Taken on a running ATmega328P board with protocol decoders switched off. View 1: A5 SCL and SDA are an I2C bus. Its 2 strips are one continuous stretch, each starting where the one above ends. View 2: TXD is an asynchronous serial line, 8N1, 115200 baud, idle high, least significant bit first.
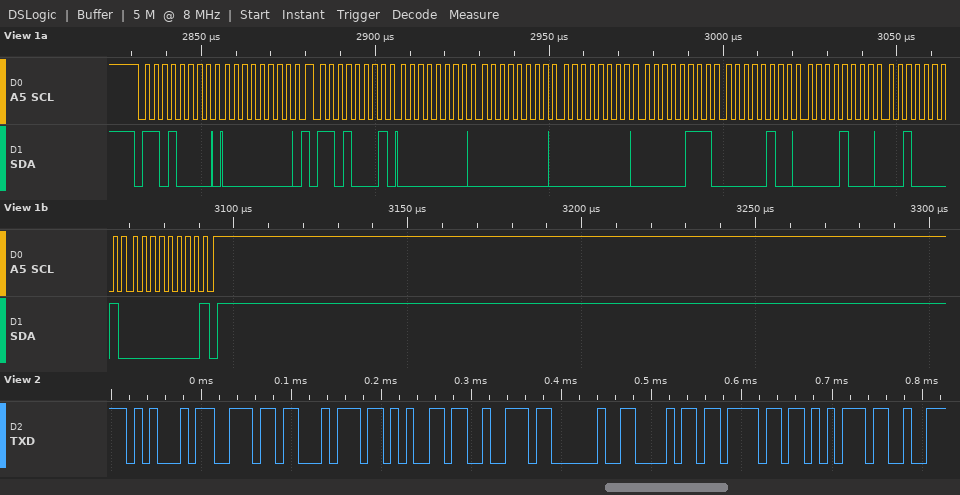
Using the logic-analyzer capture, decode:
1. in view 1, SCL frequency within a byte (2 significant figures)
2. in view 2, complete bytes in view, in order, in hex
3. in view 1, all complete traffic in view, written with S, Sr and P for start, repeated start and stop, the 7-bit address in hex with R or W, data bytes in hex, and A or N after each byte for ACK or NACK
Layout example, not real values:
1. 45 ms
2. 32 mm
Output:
1. 400 kHz
2. 45 6E 74 65 72 20 68 6F 75
3. S 68W A 00 A Sr 68R A 00 A 00 A 00 A 07 A 04 A 08 A 21 A 00 N P
